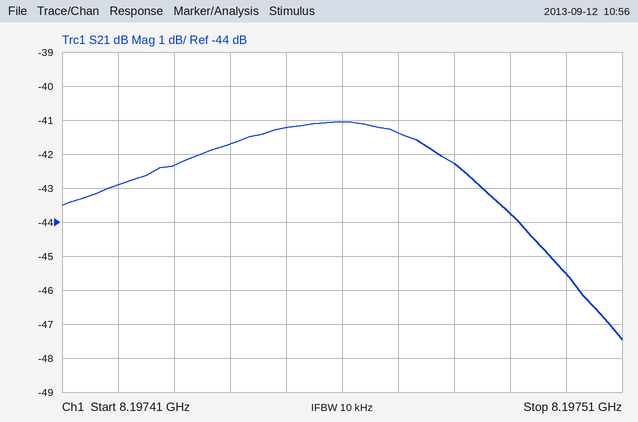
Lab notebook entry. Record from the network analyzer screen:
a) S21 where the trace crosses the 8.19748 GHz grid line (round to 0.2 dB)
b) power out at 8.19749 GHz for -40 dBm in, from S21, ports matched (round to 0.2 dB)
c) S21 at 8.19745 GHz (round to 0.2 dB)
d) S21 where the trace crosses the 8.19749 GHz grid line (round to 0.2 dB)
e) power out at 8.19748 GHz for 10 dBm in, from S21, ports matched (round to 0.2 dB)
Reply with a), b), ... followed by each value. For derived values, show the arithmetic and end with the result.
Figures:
a) -42.2 dB
b) -40 dBm + (-43.8 dB) = -83.8 dBm
c) -41.2 dB
d) -43.8 dB
e) 10 dBm + (-42.2 dB) = -32.2 dBm
